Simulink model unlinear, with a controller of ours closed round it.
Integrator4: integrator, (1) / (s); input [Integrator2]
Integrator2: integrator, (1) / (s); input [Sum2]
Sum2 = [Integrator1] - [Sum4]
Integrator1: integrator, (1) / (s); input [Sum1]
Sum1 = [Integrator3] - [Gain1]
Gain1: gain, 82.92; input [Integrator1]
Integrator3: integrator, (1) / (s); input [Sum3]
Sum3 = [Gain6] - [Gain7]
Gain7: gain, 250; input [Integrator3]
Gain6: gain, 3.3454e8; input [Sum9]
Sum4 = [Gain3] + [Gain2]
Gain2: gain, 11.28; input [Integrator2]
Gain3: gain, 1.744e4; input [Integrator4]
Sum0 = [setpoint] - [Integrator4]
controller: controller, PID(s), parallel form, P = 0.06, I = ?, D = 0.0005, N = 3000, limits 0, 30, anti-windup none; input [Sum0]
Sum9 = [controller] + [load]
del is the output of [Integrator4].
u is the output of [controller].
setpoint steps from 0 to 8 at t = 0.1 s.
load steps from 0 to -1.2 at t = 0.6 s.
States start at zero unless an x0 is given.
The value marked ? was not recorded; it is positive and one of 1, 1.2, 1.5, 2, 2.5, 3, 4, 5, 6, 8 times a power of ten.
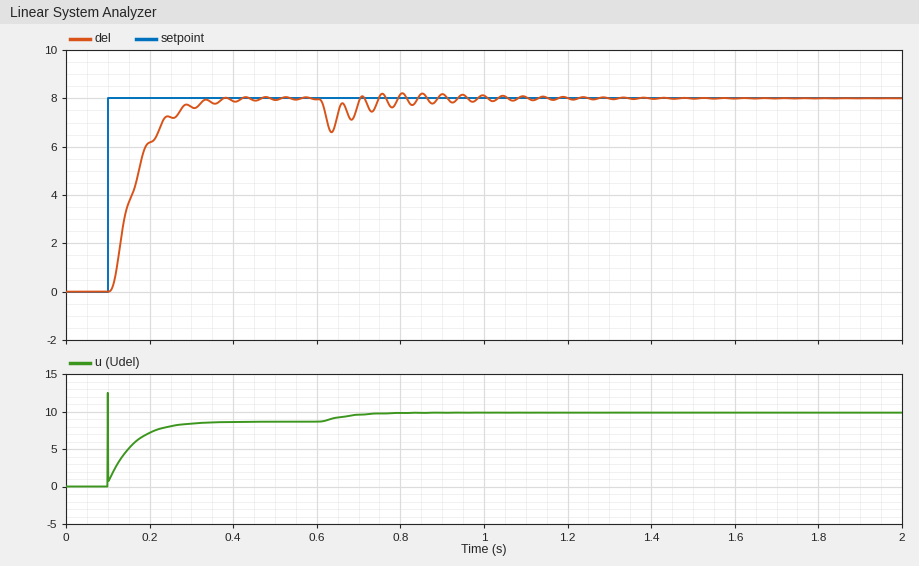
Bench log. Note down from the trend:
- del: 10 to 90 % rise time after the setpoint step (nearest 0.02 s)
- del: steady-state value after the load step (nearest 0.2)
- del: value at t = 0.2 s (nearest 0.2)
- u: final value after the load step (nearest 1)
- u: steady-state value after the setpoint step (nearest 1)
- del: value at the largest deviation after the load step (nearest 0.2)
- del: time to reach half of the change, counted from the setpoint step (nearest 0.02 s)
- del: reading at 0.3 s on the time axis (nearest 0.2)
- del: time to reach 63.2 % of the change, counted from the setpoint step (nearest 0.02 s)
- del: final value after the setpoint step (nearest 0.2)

0.12 s
8.0
6.2
10
9
6.6
0.06 s
7.6
0.08 s
8.0
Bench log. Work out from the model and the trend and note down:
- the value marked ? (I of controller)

15
